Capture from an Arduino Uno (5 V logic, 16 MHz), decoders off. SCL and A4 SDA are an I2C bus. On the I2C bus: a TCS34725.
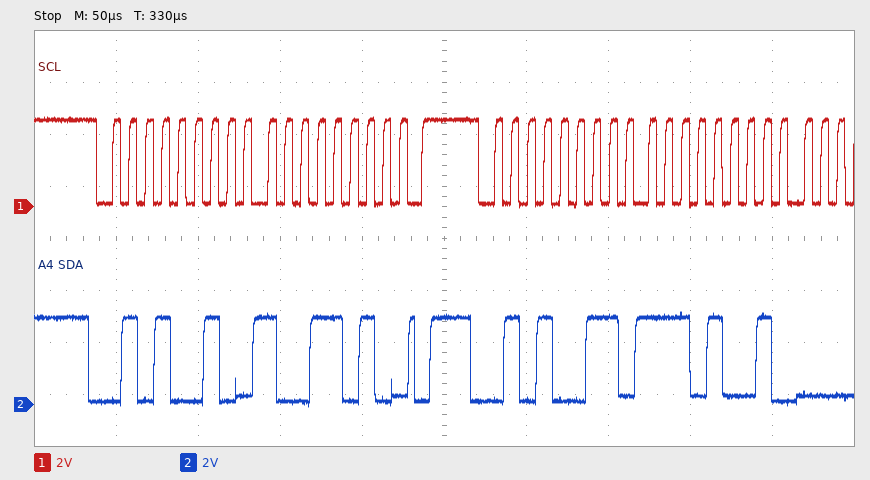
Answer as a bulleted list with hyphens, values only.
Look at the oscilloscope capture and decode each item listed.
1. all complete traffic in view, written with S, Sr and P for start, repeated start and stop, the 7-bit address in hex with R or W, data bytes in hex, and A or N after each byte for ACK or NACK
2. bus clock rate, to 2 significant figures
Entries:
- S 29W A 9A A P S 29R A E9 A
- 100 kHz
